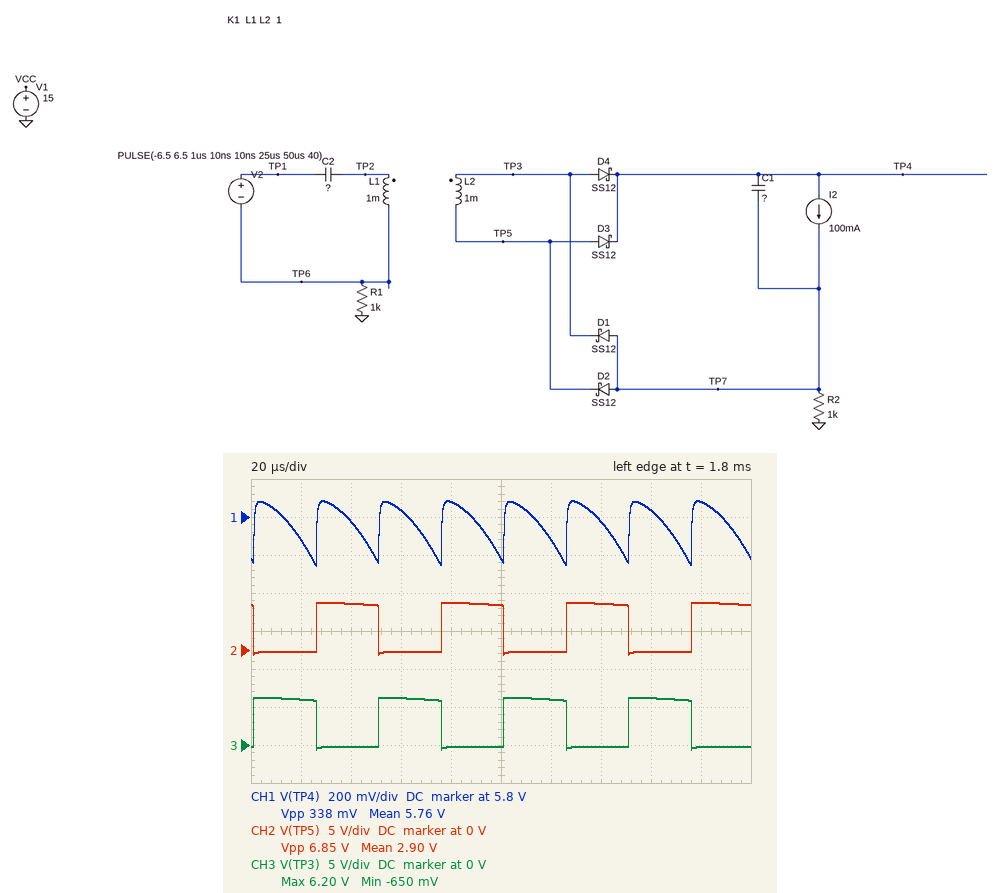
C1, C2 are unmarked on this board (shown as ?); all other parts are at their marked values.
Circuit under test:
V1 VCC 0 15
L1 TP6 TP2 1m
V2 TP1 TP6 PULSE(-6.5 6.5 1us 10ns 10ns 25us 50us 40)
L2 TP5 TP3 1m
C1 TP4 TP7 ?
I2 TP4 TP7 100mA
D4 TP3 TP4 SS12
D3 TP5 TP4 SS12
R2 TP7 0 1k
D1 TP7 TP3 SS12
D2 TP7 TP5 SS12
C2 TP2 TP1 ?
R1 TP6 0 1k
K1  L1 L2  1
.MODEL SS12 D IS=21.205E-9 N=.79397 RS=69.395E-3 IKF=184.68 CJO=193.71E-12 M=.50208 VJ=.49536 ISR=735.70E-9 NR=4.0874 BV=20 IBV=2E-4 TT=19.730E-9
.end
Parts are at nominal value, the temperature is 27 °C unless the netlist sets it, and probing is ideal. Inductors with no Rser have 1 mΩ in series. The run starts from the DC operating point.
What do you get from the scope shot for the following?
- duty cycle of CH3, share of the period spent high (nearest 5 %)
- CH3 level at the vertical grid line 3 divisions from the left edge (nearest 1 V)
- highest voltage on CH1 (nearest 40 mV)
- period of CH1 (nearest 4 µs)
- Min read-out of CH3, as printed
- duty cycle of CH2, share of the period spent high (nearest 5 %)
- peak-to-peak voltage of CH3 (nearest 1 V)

50 %
6 V
5.88 V
24 µs
-650 mV
50 %
7 V
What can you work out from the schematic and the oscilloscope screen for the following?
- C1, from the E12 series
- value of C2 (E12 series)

3.3 µF
3.3 µF
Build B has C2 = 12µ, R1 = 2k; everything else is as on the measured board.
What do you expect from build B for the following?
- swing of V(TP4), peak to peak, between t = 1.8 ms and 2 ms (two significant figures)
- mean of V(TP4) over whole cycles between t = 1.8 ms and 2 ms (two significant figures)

140 mV
5.9 V
